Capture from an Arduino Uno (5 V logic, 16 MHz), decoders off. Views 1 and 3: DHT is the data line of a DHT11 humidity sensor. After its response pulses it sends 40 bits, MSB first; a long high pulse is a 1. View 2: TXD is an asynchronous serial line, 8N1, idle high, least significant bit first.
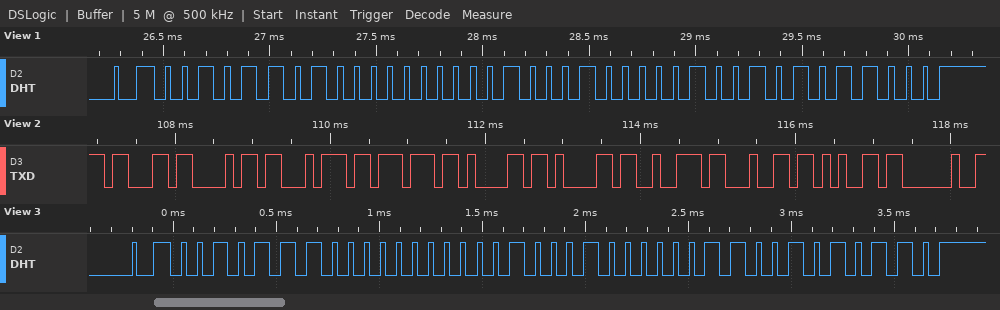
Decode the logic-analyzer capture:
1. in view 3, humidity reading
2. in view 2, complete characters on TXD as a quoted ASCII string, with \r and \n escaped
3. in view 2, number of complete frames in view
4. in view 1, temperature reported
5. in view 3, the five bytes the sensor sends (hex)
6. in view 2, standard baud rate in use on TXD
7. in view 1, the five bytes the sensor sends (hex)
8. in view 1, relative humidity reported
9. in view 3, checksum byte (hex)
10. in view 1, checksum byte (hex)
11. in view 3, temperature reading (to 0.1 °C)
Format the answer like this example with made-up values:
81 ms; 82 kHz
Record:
46 %; "chtwaarde "; 10; 34.9 °C; 2E 00 22 06 56; 9600 baud; 2D 00 22 09 58; 45 %; 0x56; 0x58; 34.6 °C
